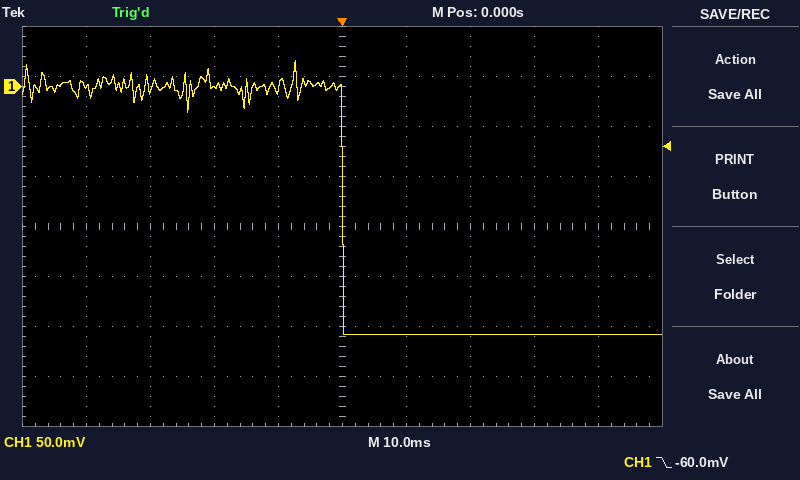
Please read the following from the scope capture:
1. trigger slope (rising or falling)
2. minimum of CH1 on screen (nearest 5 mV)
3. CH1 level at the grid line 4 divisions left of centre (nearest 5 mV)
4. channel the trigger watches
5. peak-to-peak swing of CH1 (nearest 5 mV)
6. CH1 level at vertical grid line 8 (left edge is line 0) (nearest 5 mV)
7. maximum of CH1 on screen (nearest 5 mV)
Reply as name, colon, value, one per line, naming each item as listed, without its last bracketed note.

trigger slope: falling
minimum of CH1 on screen: -250 mV
CH1 level at the grid line 4 divisions left of centre: 0 mV
channel the trigger watches: CH1
peak-to-peak swing of CH1: 275 mV
CH1 level at vertical grid line 8 (left edge is line 0): -250 mV
maximum of CH1 on screen: 25 mV
